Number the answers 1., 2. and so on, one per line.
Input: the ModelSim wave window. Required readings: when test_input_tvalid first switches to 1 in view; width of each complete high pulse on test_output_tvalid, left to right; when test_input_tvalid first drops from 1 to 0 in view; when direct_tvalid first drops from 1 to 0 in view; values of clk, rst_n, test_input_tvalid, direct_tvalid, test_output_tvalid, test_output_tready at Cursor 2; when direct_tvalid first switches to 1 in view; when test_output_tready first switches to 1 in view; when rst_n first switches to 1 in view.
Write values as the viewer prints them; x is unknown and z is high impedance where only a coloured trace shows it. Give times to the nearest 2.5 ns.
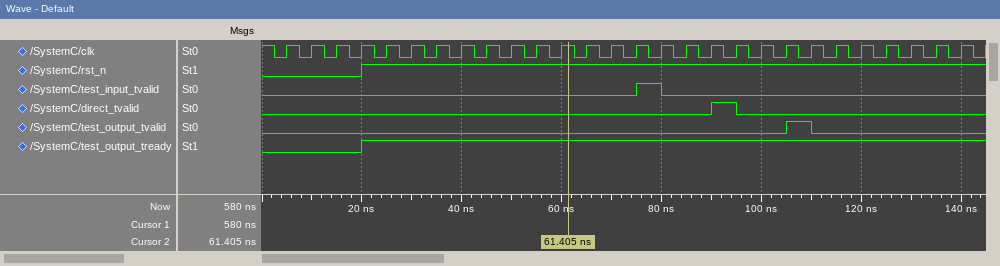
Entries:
1. 75 ns
2. 5 ns
3. 80 ns
4. 95 ns
5. clk=1, rst_n=1, test_input_tvalid=0, direct_tvalid=0, test_output_tvalid=0, test_output_tready=1
6. 90 ns
7. 20 ns
8. 20 ns
